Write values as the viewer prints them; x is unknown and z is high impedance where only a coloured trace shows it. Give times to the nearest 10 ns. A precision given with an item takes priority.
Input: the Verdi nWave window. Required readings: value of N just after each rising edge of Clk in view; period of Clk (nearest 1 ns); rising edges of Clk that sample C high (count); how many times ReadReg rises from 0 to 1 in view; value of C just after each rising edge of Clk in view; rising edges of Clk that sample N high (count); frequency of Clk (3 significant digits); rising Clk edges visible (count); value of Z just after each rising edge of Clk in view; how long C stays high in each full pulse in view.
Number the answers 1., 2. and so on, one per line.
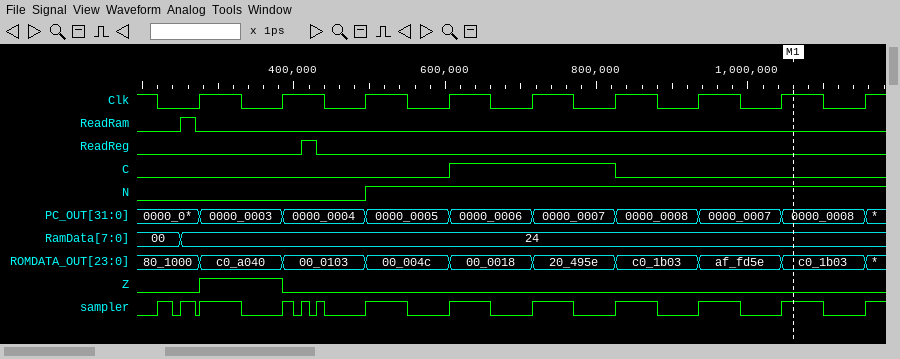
1. 0 0 1 1 1 1 1 1 1
2. 110 ns
3. 2
4. 1
5. 0 0 0 1 1 0 0 0 0
6. 6
7. 9.09 MHz
8. 9
9. 1 0 0 0 0 0 0 0 0
10. 220 ns
